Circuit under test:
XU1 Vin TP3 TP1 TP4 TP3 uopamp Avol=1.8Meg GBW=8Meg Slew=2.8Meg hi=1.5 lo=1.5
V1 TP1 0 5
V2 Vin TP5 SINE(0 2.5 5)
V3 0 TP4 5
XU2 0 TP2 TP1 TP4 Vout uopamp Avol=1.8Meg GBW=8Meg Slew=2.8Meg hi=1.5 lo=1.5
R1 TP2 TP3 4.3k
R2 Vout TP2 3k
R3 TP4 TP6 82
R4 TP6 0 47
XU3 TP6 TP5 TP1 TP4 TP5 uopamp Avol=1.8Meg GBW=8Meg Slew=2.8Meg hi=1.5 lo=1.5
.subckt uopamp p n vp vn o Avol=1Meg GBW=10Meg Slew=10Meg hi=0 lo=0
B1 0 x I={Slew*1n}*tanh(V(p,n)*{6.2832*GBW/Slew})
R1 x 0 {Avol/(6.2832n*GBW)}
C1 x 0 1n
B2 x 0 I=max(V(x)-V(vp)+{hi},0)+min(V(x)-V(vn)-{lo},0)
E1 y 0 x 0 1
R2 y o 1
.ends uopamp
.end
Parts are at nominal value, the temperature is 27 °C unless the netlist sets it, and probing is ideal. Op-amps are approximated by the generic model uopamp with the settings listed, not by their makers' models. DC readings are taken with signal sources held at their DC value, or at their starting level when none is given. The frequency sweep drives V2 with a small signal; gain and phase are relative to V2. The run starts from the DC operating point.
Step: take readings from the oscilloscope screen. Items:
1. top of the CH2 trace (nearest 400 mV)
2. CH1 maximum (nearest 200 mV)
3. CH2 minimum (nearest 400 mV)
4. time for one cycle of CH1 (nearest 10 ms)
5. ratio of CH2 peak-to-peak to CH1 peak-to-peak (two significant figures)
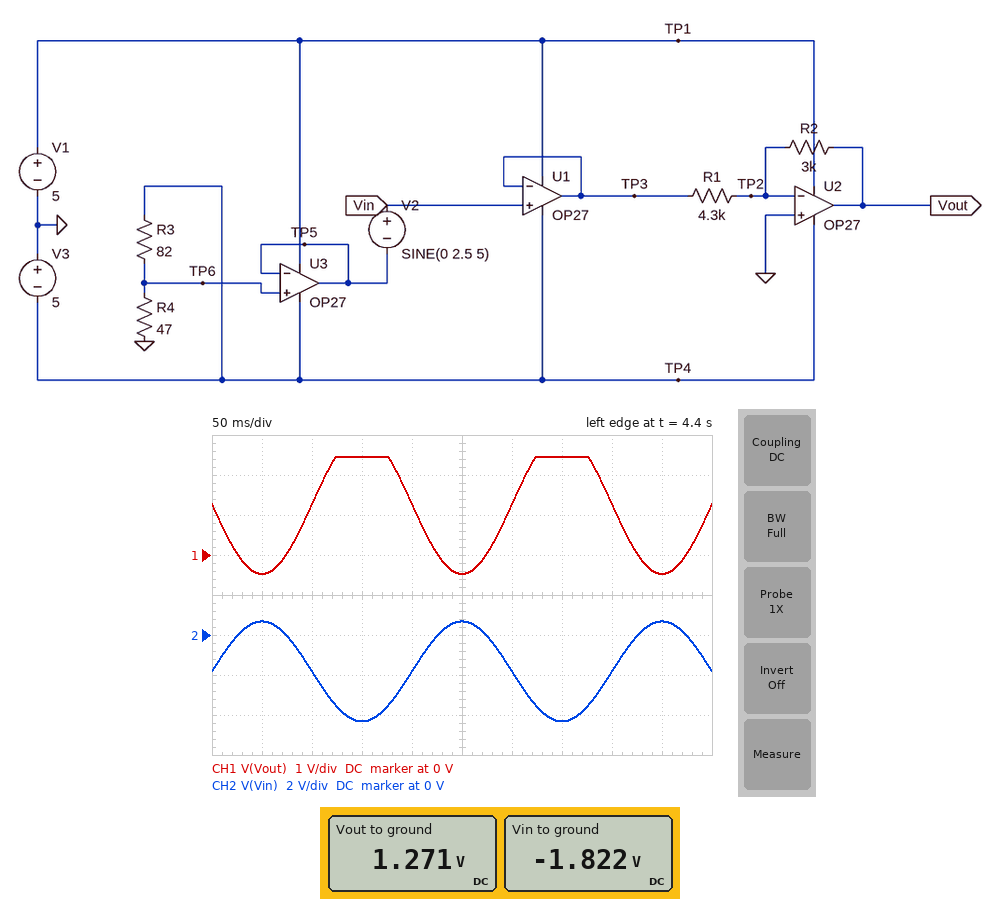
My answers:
800 mV
2.4 V
-4.4 V
200 ms
1.7
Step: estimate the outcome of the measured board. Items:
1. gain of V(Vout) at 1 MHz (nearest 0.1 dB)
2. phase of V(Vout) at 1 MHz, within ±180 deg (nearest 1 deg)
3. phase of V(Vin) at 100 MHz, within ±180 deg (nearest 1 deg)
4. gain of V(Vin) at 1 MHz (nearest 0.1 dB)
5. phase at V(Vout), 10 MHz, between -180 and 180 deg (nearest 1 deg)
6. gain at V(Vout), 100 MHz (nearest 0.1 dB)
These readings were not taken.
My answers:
-3.4 dB
161 deg
0 deg
0 dB
64 deg
-51.6 dB
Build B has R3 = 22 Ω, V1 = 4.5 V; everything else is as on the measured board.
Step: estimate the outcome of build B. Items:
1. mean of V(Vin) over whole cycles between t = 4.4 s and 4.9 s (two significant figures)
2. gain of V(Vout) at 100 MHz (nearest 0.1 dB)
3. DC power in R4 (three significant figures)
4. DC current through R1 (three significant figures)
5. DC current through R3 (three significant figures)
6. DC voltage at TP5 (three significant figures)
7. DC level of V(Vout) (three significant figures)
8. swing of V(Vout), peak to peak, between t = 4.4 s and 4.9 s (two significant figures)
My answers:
-3.4 V
-51.6 dB
247 mW
792 µA
72.5 mA
-3.41 V
2.38 V
1.8 V
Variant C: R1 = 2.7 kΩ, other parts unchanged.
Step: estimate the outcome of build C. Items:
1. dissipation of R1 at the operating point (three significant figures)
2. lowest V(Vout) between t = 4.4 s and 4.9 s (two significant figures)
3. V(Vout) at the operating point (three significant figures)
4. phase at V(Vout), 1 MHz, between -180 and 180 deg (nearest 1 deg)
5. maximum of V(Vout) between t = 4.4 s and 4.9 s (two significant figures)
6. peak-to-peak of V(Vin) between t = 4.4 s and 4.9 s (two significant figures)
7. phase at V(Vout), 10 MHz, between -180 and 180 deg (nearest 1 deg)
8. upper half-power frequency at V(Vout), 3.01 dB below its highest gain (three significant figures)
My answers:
1.23 mW
-750 mV
2.02 V
158 deg
3.5 V
5.0 V
59 deg
3.22 MHz
